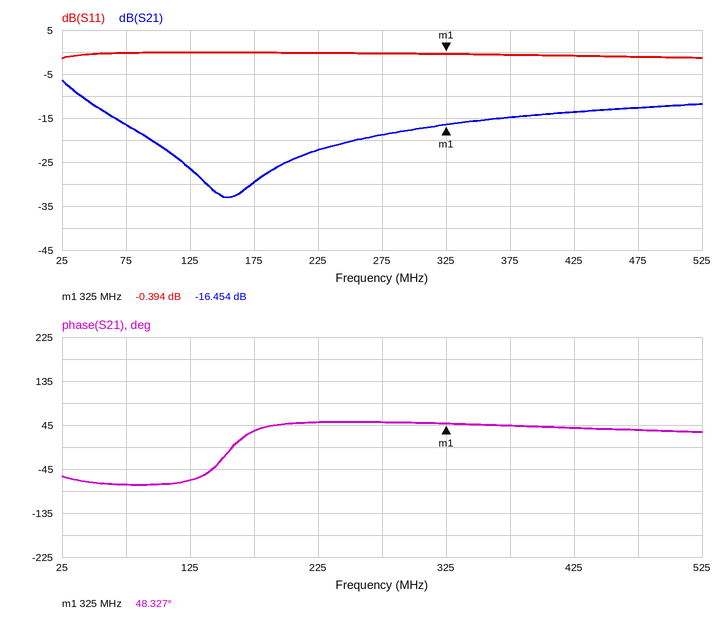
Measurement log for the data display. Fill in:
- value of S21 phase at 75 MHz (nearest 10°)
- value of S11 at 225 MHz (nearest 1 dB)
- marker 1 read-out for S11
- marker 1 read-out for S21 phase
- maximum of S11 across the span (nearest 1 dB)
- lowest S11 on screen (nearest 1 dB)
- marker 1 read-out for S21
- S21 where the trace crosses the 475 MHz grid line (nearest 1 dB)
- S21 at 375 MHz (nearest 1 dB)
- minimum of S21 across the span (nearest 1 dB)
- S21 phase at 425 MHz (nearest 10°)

-80°
0 dB
-0.394 dB
48.327°
0 dB
-1 dB
-16.454 dB
-13 dB
-15 dB
-33 dB
40°
